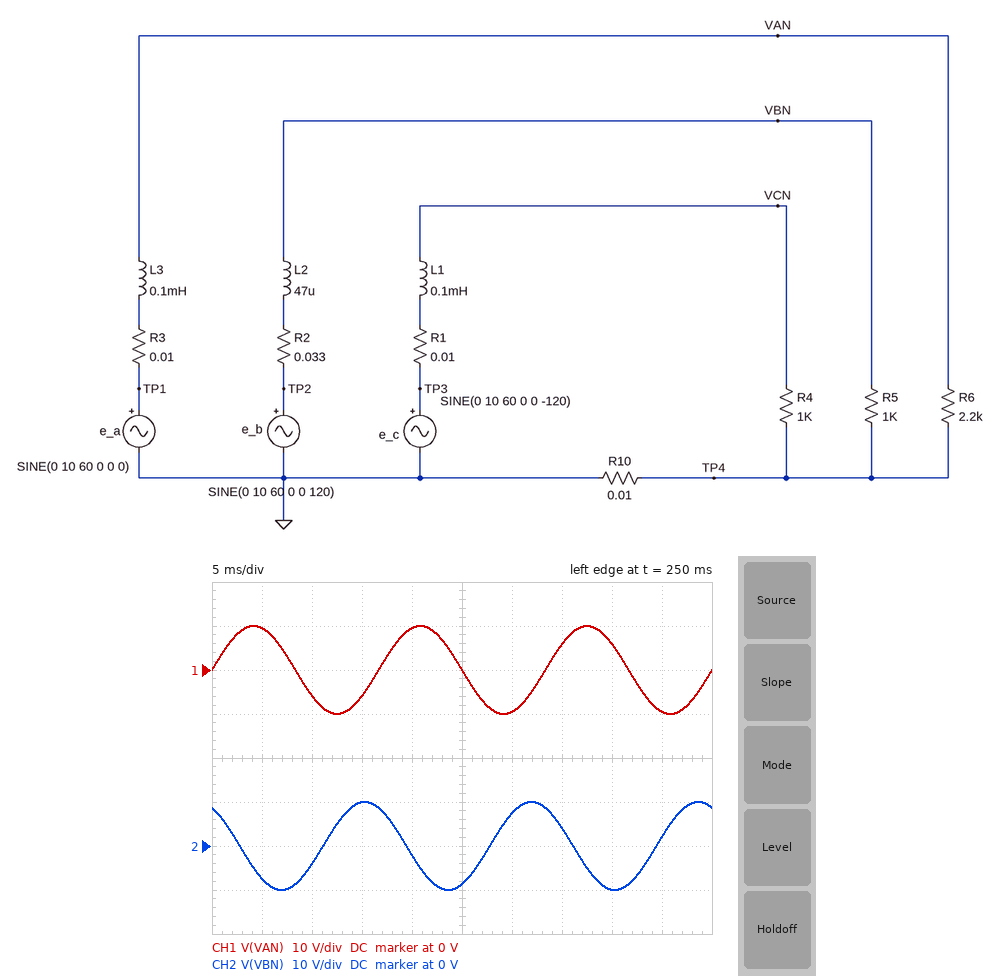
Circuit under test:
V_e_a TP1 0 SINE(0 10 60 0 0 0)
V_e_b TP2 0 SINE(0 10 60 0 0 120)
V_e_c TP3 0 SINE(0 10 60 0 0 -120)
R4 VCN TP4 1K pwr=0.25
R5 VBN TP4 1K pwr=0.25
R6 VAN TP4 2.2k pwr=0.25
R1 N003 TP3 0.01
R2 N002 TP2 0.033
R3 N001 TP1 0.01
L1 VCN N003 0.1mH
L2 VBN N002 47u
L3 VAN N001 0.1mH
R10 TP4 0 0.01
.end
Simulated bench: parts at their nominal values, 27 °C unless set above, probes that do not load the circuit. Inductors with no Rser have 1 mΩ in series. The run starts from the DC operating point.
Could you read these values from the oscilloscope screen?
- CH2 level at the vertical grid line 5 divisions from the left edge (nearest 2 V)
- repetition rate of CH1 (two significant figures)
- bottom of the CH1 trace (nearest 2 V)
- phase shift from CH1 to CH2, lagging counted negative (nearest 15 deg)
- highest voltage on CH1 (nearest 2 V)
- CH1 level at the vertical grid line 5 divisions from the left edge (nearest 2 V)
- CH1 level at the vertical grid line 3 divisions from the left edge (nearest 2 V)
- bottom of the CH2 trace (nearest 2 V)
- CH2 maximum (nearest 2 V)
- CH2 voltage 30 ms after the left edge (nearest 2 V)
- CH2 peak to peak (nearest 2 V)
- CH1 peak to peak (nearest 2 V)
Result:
-8 V
60 Hz
-10 V
120 deg
10 V
0 V
-6 V
-10 V
10 V
8 V
20 V
20 V
